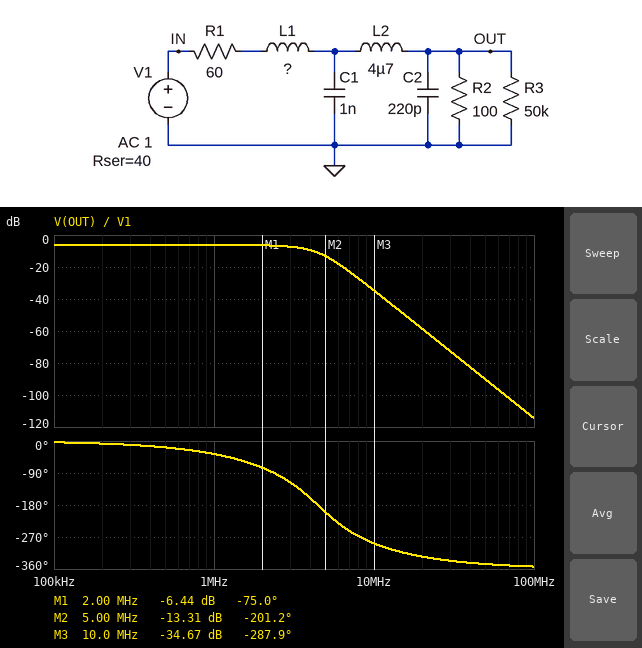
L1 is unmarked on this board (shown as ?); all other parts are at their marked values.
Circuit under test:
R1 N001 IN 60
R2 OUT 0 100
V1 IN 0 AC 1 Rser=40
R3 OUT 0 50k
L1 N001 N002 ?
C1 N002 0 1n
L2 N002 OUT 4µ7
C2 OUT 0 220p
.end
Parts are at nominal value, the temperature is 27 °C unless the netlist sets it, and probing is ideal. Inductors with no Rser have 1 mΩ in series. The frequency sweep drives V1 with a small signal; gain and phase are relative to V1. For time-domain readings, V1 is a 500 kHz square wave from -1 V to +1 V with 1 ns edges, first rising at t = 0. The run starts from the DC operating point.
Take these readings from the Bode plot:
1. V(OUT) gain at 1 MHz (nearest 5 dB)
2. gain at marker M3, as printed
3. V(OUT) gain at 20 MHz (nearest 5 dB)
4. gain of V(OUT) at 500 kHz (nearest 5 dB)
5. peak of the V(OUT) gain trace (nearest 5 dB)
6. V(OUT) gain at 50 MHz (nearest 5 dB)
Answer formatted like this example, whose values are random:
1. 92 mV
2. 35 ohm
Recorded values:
1. -5 dB
2. -34.67 dB
3. -60 dB
4. -5 dB
5. -5 dB
6. -90 dB
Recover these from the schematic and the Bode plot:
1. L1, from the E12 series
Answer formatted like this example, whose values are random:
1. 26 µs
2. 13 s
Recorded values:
1. 3.3 µH
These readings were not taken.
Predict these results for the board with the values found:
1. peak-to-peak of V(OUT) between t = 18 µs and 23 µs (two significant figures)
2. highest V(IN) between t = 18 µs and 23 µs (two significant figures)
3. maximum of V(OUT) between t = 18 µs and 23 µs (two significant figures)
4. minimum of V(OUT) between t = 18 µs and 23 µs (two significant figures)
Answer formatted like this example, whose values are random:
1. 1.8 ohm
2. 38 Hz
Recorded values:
1. 1.1 V
2. 1.2 V
3. 560 mV
4. -560 mV
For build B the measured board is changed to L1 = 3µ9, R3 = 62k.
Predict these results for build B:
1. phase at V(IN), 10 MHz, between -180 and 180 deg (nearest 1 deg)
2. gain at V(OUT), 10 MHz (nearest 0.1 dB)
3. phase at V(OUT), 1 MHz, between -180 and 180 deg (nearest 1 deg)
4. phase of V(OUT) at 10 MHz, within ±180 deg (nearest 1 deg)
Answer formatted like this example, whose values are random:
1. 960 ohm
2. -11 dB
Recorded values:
1. 9 deg
2. -35.9 dB
3. -38 deg
4. 68 deg
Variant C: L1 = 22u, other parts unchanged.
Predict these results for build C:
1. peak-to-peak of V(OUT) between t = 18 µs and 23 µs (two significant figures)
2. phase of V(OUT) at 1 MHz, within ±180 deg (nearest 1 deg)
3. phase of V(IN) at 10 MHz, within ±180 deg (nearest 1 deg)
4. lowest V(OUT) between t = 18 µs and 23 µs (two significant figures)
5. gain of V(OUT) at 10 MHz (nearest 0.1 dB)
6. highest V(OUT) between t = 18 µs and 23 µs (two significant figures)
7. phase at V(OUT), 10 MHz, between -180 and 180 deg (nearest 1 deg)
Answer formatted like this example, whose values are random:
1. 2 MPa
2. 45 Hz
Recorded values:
1. 1.0 V
2. -71 deg
3. 2 deg
4. -510 mV
5. -50.7 dB
6. 510 mV
7. 49 deg
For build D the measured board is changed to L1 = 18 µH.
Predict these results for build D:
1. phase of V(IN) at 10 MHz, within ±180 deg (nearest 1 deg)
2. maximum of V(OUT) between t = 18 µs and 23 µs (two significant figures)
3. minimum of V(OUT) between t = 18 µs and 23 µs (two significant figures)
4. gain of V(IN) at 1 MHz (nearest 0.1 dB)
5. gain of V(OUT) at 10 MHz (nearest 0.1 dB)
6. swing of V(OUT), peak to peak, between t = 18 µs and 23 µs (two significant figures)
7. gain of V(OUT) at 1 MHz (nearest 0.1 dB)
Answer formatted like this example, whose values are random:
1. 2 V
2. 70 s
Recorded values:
1. 2 deg
2. 520 mV
3. -520 mV
4. -1.8 dB
5. -49.0 dB
6. 1.0 V
7. -6.7 dB
